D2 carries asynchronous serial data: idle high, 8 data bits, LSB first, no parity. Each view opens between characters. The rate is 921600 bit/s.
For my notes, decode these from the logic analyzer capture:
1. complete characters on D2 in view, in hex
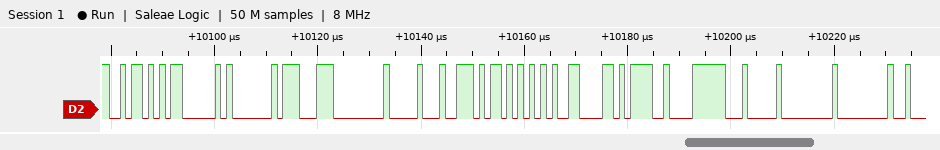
5A, 03, 01, C7, 00, 10, AE, 55, 86, 3D, F8, 04, 00, 00
